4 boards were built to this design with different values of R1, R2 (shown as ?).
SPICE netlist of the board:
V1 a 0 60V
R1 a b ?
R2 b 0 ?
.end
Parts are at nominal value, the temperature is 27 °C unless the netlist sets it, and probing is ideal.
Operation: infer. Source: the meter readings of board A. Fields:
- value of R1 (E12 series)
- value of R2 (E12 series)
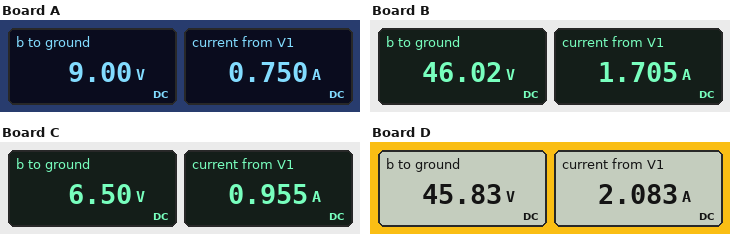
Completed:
68 Ω
12 Ω
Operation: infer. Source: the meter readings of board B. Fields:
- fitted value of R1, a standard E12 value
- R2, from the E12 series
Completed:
8.2 Ω
27 Ω
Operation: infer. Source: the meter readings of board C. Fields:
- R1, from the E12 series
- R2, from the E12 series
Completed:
56 Ω
6.8 Ω
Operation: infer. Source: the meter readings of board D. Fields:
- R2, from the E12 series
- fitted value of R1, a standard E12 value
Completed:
22 Ω
6.8 Ω
